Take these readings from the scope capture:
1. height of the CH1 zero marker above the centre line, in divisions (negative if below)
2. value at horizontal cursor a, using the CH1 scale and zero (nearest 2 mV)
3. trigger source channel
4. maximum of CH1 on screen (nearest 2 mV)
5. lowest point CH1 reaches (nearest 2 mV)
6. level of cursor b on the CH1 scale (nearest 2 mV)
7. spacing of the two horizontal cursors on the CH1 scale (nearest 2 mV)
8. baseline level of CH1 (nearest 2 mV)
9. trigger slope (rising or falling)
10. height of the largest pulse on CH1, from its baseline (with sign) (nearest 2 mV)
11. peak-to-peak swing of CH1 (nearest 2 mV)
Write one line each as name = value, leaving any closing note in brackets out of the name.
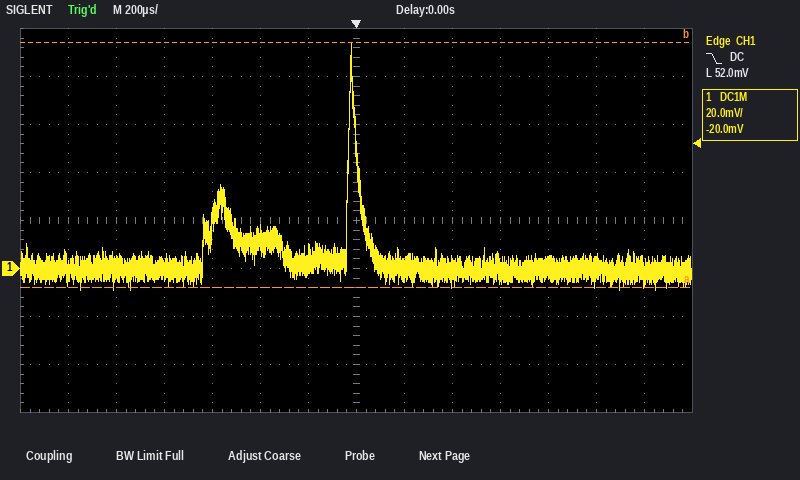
height of the CH1 zero marker above the centre line, in divisions = -1.0 div
value at horizontal cursor a, using the CH1 scale and zero = -8 mV
trigger source channel = CH1
maximum of CH1 on screen = 94 mV
lowest point CH1 reaches = -8 mV
level of cursor b on the CH1 scale = 94 mV
spacing of the two horizontal cursors on the CH1 scale = 102 mV
baseline level of CH1 = 0 mV
trigger slope = falling
height of the largest pulse on CH1, from its baseline (with sign) = +94 mV
peak-to-peak swing of CH1 = 102 mV
